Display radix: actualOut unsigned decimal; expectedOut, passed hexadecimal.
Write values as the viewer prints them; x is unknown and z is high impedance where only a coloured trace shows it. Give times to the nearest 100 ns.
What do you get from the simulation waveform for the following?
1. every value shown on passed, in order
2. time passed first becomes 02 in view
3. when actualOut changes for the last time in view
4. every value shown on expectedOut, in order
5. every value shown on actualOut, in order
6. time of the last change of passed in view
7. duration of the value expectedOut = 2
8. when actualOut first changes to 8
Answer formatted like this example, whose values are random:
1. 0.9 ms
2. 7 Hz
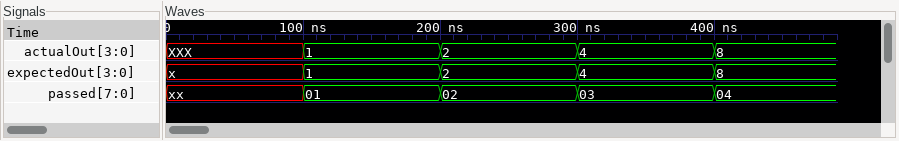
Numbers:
1. xx, 01, 02, 03, 04
2. 200 ns
3. 400 ns
4. x, 1, 2, 4, 8
5. XXX, 1, 2, 4, 8
6. 400 ns
7. 100 ns
8. 400 ns
